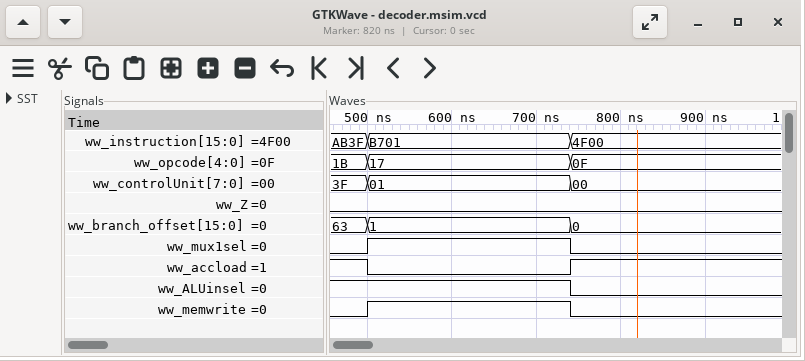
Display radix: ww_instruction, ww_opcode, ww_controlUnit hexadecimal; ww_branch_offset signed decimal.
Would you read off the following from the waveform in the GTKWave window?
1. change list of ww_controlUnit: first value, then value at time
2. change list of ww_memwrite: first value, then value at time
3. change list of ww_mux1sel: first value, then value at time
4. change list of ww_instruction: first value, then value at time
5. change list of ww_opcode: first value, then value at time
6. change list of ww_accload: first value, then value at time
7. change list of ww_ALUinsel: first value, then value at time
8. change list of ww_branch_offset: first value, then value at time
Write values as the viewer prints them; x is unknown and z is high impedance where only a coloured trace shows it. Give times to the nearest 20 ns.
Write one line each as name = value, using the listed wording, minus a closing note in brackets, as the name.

change list of ww_controlUnit: first value, then value at time = 3F, 01 at 500 ns, 00 at 740 ns
change list of ww_memwrite: first value, then value at time = 0, 1 at 500 ns, 0 at 740 ns
change list of ww_mux1sel: first value, then value at time = 0, 1 at 500 ns, 0 at 740 ns
change list of ww_instruction: first value, then value at time = AB3F, B701 at 500 ns, 4F00 at 740 ns
change list of ww_opcode: first value, then value at time = 1B, 17 at 500 ns, 0F at 740 ns
change list of ww_accload: first value, then value at time = 1, 0 at 500 ns, 1 at 740 ns
change list of ww_ALUinsel: first value, then value at time = 1, 0 at 740 ns
change list of ww_branch_offset: first value, then value at time = 63, 1 at 500 ns, 0 at 740 ns
